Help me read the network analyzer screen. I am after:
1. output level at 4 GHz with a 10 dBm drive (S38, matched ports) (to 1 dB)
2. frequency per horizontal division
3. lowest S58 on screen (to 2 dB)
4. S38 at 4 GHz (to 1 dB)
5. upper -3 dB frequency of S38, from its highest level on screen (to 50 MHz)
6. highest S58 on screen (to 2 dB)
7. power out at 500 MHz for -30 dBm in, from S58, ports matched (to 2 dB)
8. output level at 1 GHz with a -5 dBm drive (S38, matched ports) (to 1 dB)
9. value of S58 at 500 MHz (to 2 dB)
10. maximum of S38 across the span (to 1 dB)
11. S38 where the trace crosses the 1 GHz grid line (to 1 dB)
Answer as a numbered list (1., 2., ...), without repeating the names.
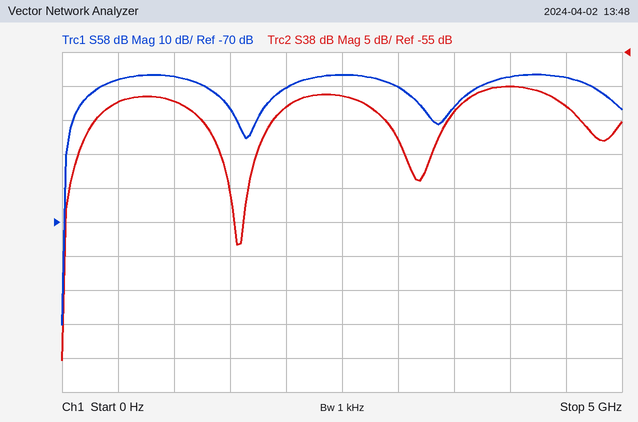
1. -50 dBm
2. 500 MHz
3. -100 dB
4. -60 dB
5. 4.50 GHz
6. -26 dB
7. -58 dBm
8. -67 dBm
9. -28 dB
10. -60 dB
11. -62 dB
